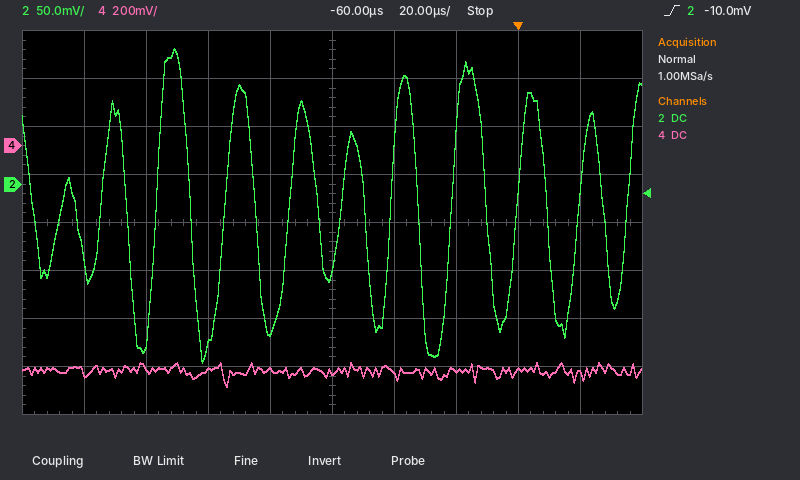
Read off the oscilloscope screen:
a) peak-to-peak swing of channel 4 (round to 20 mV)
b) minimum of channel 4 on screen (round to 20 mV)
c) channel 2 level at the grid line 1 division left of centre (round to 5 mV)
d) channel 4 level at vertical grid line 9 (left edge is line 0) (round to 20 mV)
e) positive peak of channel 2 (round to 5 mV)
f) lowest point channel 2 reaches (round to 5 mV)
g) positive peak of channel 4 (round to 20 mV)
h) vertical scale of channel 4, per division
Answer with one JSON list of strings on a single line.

["100 mV", "-1.00 V", "-155 mV", "-960 mV", "140 mV", "-185 mV", "-900 mV", "200 mV"]
